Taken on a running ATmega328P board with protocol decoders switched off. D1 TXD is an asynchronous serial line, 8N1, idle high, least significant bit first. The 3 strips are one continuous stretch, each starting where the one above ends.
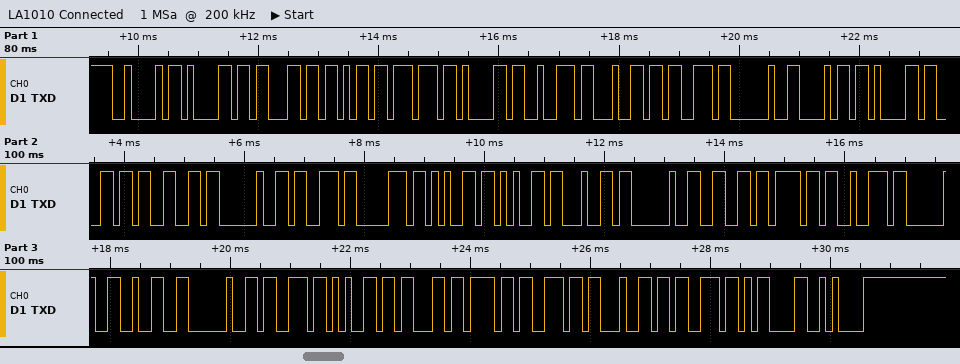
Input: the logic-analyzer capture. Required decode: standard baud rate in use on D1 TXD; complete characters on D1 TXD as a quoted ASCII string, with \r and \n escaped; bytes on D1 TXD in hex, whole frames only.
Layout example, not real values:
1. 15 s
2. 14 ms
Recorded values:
1. 9600 baud
2. "Backwards half speed for 2 seconds\r\n"
3. 0x42 0x61 0x63 0x6B 0x77 0x61 0x72 0x64 0x73 0x20 0x68 0x61 0x6C 0x66 0x20 0x73 0x70 0x65 0x65 0x64 0x20 0x66 0x6F 0x72 0x20 0x32 0x20 0x73 0x65 0x63 0x6F 0x6E 0x64 0x73 0x0D 0x0A
